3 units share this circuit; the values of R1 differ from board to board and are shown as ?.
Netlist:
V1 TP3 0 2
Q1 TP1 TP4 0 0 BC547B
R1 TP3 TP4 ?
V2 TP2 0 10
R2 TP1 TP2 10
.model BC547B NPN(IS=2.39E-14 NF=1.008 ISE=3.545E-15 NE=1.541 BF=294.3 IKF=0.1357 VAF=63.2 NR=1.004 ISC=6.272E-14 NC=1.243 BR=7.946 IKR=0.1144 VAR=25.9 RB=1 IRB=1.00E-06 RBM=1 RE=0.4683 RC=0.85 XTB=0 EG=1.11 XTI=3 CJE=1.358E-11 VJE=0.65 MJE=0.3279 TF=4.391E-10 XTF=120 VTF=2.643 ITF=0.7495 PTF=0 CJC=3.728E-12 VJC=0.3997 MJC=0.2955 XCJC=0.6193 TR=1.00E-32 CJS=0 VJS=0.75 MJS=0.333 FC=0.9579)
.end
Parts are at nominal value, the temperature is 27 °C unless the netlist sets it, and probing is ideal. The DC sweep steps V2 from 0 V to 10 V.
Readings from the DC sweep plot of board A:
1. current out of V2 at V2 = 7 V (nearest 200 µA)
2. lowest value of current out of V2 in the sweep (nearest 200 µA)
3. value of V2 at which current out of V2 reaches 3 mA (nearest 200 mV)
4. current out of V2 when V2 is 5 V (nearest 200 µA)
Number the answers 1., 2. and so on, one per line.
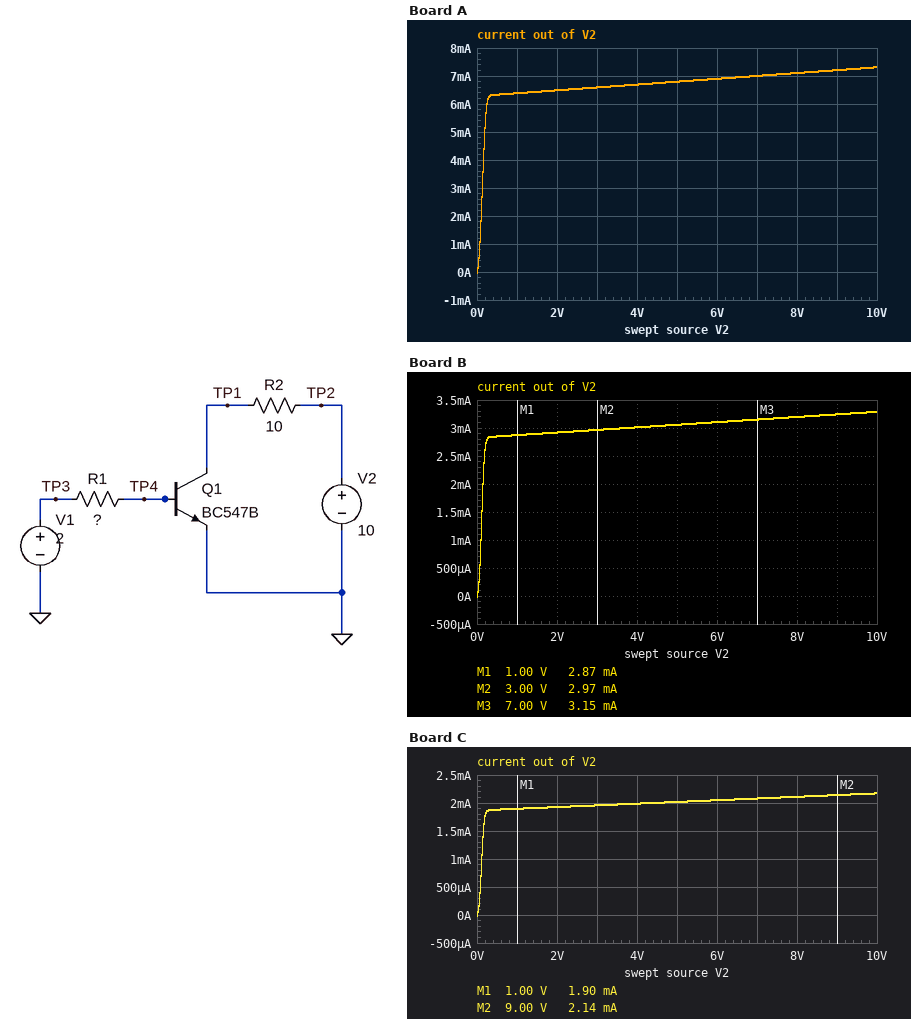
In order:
1. 7.0 mA
2. 0 A
3. 200 mV
4. 6.8 mA
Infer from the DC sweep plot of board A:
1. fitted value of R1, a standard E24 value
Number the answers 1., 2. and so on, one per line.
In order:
1. 56 kΩ
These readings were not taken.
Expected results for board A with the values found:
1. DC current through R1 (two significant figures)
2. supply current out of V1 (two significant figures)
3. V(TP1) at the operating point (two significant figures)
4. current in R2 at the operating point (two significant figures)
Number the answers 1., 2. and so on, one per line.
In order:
1. 23 µA
2. 23 µA
3. 9.9 V
4. 7.3 mA
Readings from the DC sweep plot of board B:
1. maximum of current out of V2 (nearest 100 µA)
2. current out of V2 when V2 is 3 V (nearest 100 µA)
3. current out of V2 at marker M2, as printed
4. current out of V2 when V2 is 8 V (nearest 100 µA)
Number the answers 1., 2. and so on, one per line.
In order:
1. 3.3 mA
2. 3.0 mA
3. 2.97 mA
4. 3.2 mA
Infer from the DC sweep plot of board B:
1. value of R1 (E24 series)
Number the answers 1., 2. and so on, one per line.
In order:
1. 130 kΩ
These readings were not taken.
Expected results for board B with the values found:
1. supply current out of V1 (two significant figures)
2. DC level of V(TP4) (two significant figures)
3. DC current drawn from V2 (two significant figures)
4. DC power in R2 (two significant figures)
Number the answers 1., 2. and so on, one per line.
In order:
1. 10 µA
2. 670 mV
3. 3.3 mA
4. 110 µW
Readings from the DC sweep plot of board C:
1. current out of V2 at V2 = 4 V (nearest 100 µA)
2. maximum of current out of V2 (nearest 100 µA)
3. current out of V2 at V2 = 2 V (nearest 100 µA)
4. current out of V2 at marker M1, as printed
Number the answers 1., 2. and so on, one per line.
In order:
1. 2.0 mA
2. 2.2 mA
3. 1.9 mA
4. 1.90 mA
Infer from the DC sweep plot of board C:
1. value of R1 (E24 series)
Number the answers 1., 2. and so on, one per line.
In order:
1. 200 kΩ
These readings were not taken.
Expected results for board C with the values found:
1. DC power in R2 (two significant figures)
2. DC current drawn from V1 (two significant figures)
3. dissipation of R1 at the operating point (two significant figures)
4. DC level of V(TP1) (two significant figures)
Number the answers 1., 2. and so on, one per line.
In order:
1. 47 µW
2. 6.7 µA
3. 9.0 µW
4. 10 V
